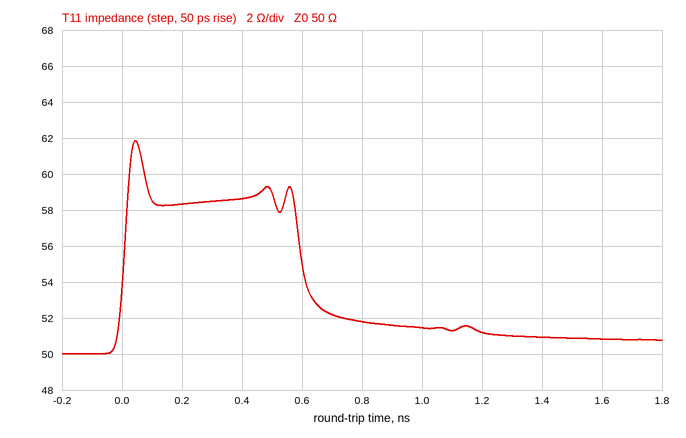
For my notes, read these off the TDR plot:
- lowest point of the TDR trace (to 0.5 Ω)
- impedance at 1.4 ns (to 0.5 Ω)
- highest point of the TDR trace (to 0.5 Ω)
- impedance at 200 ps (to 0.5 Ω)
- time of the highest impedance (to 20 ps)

50.0 Ω
51.0 Ω
62.0 Ω
58.5 Ω
40 ps
